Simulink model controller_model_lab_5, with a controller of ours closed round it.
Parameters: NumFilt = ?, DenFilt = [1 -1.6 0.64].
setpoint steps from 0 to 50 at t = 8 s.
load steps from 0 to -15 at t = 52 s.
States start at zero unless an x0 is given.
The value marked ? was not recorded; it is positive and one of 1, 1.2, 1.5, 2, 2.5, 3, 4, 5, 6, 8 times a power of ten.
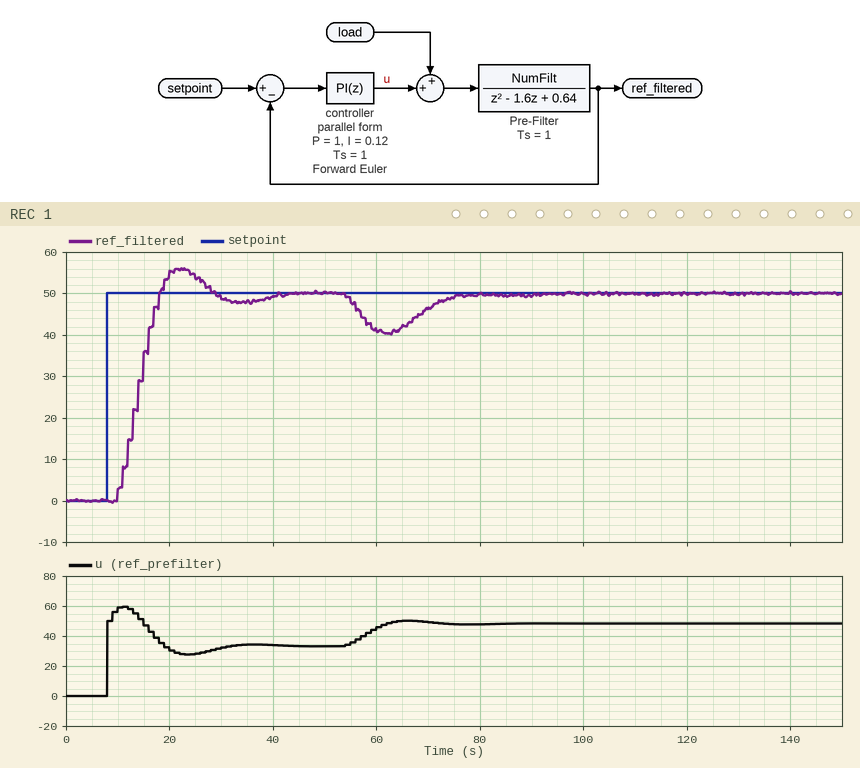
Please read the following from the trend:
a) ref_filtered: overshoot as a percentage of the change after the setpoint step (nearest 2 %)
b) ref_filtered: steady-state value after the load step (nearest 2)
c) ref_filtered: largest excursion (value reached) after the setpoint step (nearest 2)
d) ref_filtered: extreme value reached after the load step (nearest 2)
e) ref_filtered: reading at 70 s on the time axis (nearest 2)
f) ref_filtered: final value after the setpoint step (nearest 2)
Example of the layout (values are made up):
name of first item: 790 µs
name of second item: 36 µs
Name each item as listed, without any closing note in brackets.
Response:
ref_filtered: overshoot as a percentage of the change after the setpoint step: 12 %
ref_filtered: steady-state value after the load step: 50
ref_filtered: largest excursion (value reached) after the setpoint step: 56
ref_filtered: extreme value reached after the load step: 40
ref_filtered: reading at 70 s on the time axis: 46
ref_filtered: final value after the setpoint step: 50
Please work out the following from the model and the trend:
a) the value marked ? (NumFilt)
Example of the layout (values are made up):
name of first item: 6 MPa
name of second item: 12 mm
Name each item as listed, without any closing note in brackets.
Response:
the value marked ?: 0.06
